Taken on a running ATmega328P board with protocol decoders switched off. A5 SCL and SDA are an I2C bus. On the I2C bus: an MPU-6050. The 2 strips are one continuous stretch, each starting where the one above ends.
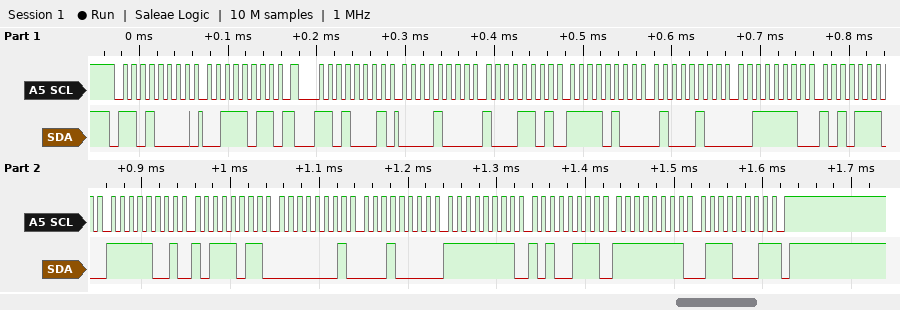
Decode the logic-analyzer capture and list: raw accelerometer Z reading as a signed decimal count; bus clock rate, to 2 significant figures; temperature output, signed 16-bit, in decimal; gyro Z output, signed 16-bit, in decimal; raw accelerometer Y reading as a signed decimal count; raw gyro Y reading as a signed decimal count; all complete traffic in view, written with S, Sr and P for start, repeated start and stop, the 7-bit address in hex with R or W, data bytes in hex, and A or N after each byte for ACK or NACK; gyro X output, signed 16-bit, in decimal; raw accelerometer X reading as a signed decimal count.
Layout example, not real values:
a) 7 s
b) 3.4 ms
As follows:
a) 16046
b) 100 kHz
c) -1605
d) -143
e) -3004
f) -89
g) S 68W A 3B A Sr 68R A 08 A 8D A F4 A 44 A 3E A AE A F9 A BB A 01 A 10 A FF A A7 A FF A 71 N P
h) 272
i) 2189
